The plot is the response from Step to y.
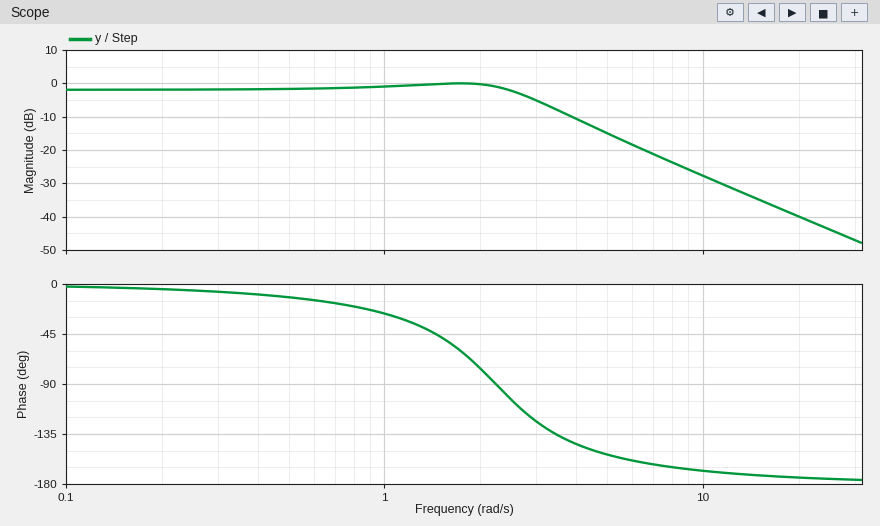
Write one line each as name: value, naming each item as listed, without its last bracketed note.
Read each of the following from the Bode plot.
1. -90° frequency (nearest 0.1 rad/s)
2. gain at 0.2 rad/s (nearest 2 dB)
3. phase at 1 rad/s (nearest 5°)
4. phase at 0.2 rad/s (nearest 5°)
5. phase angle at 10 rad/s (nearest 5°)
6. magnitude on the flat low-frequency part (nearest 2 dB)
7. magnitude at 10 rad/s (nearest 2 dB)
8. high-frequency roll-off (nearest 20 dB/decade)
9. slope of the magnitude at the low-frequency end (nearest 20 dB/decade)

-90° frequency: 2.2 rad/s
gain at 0.2 rad/s: -2 dB
phase at 1 rad/s: -25°
phase at 0.2 rad/s: -5°
phase angle at 10 rad/s: -170°
magnitude on the flat low-frequency part: -2 dB
magnitude at 10 rad/s: -28 dB
high-frequency roll-off: -40 dB/decade
slope of the magnitude at the low-frequency end: 0 dB/decade
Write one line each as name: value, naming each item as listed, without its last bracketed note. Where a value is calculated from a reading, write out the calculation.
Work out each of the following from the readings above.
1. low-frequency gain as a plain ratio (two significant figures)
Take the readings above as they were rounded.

low-frequency gain as a plain ratio: 10^(-2 / 20) = 0.79
